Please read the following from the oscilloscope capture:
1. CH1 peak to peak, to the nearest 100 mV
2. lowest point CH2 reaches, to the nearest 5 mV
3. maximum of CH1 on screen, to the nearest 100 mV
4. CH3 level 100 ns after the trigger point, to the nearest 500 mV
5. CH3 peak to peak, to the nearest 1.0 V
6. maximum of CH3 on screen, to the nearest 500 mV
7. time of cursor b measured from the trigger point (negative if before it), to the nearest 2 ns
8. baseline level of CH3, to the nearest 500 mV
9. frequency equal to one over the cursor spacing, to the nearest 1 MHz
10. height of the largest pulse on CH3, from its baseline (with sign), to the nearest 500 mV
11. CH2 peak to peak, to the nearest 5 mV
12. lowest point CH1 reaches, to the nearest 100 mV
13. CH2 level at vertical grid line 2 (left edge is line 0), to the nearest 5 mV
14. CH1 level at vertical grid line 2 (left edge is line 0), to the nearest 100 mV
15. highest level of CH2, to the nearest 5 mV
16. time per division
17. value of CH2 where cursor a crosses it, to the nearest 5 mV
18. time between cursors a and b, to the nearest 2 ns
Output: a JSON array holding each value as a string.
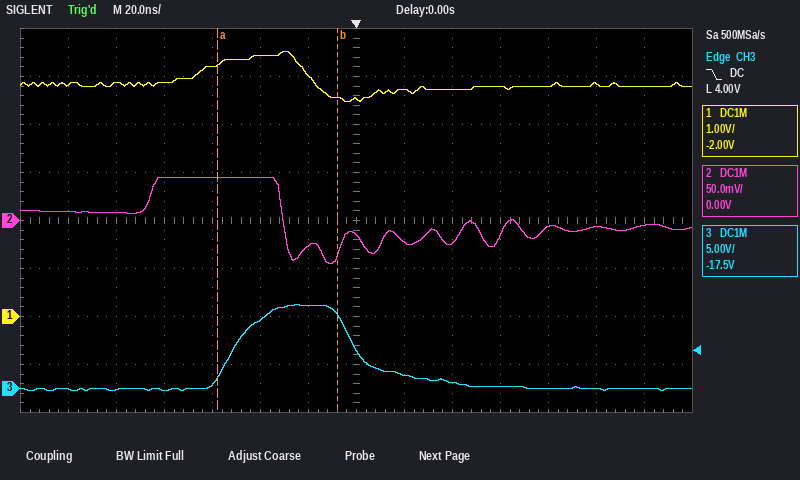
["1.0 V", "-45 mV", "5.5 V", "0.0 V", "9.0 V", "9.0 V", "-8 ns", "0.0 V", "20 MHz", "+9.0 V", "90 mV", "4.5 V", "10 mV", "4.9 V", "45 mV", "20 ns", "45 mV", "50 ns"]
